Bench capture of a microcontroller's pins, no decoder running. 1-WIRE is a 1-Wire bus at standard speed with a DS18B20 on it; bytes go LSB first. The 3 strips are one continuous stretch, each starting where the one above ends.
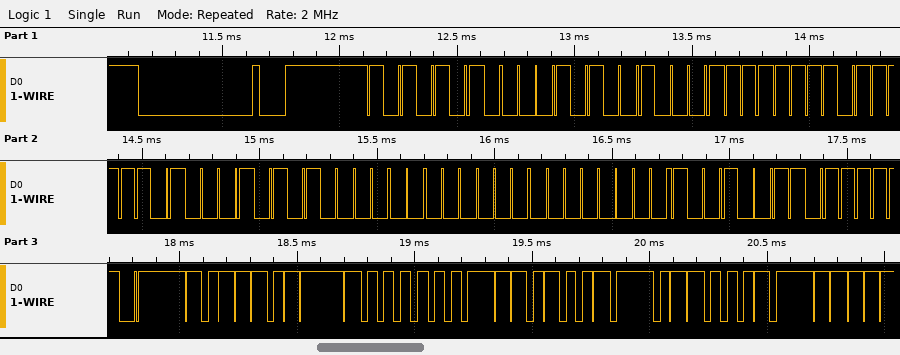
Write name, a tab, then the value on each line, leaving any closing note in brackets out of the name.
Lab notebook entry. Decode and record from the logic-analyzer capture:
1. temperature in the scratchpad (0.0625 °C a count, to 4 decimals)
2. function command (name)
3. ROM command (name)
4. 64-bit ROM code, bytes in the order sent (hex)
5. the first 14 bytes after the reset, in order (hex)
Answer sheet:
temperature in the scratchpad	29.8125 °C
function command	Read Scratchpad
ROM command	Match ROM
64-bit ROM code, bytes in the order sent	28 F1 EF 8B 0A 00 00 C9
the first 14 bytes after the reset, in order	55 28 F1 EF 8B 0A 00 00 C9 BE DD 01 4B 46
